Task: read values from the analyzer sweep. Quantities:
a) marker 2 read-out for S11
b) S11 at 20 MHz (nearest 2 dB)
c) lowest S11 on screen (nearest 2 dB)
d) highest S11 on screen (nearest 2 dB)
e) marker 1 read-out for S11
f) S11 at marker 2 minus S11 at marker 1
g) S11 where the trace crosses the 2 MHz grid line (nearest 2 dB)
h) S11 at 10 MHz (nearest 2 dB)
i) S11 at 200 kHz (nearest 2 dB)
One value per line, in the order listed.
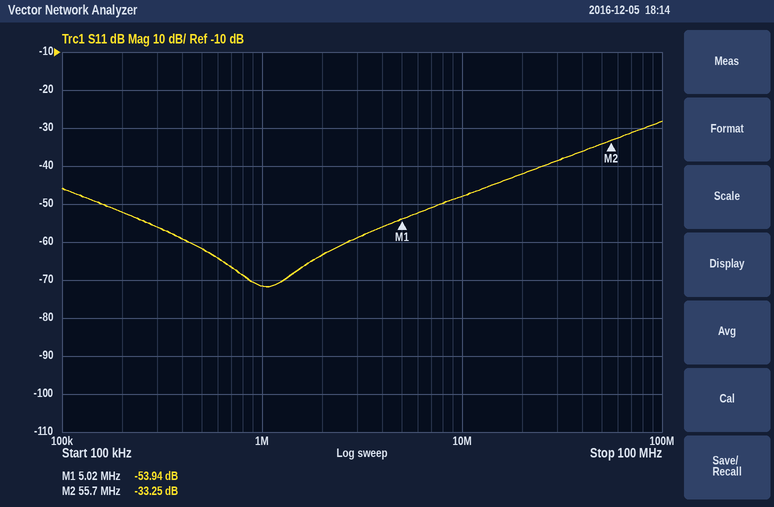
-33.25 dB
-42 dB
-72 dB
-28 dB
-53.94 dB
20.69 dB
-64 dB
-48 dB
-52 dB
